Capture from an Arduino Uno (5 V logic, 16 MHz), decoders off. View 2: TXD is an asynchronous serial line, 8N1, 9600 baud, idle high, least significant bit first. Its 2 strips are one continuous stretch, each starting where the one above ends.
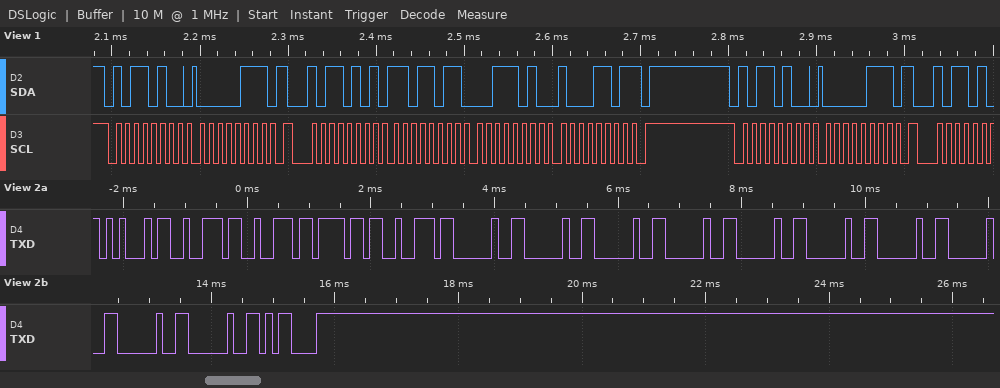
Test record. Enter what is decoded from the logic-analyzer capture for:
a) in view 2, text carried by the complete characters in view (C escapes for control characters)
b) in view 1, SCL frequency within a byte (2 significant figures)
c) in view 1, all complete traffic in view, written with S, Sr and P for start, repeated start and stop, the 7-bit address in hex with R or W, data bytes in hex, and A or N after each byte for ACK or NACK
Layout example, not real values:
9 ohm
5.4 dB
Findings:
"Error          \r"
100 kHz
S 5AW A 07 A Sr 5AR A DB A 3A A 8D N P S 5AW A 07 A
